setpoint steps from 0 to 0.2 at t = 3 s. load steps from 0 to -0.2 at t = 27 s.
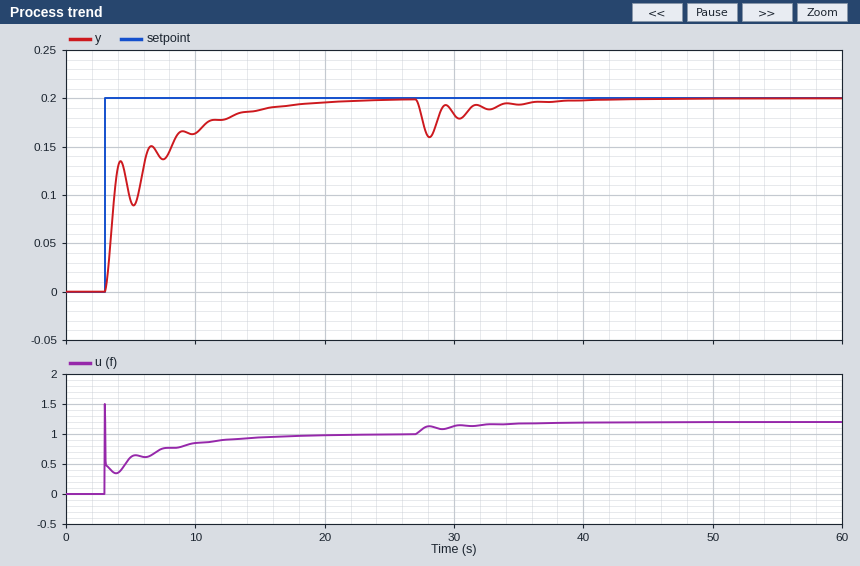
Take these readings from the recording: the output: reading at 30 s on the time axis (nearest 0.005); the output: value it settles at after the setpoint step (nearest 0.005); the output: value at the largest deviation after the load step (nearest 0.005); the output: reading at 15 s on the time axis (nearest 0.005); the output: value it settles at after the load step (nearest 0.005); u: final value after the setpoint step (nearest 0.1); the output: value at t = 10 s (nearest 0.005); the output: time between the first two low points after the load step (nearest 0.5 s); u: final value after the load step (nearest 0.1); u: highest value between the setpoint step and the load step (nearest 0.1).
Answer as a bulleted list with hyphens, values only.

- 0.185
- 0.200
- 0.160
- 0.190
- 0.200
- 1.0
- 0.165
- 2.5 s
- 1.2
- 1.5
